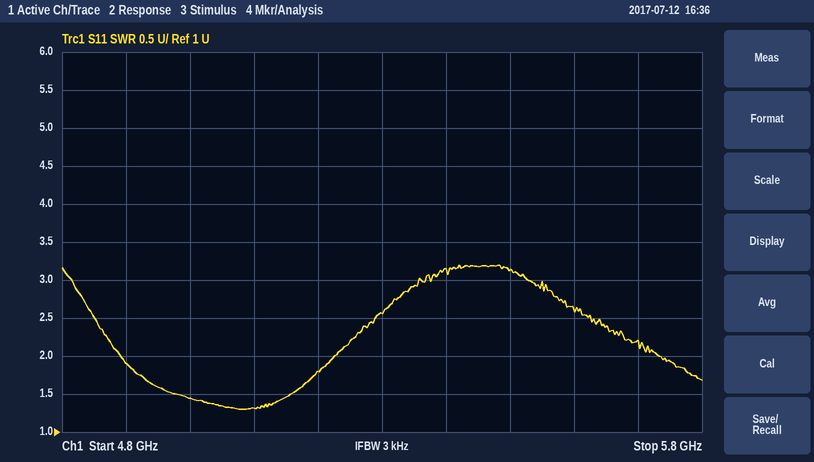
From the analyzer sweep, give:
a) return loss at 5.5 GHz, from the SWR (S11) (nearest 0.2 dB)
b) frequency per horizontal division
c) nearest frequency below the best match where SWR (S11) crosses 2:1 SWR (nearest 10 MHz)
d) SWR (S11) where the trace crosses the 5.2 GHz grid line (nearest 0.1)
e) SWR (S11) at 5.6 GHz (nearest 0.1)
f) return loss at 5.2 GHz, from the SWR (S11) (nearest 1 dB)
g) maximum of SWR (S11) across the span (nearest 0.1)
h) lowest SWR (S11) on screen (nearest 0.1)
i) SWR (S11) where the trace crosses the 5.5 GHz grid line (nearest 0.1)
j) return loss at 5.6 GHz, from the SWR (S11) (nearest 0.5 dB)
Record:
5.8 dB
100 MHz
4.89 GHz
1.8
2.6
11 dB
3.2
1.3
3.1
7.0 dB
